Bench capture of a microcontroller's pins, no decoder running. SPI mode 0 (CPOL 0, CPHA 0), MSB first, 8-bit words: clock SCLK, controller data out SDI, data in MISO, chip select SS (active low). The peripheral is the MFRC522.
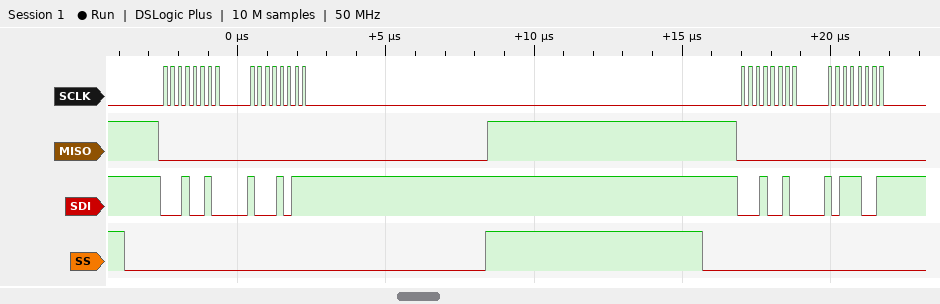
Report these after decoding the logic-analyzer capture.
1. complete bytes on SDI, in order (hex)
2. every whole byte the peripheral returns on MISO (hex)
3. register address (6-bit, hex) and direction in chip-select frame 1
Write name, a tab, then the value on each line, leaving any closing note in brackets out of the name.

complete bytes on SDI, in order	0x12 0x8B 0x12 0xB9
every whole byte the peripheral returns on MISO	0x00 0x00 0x00 0x00
register address (6-bit, hex) and direction in chip-select frame 1	0x09 write
